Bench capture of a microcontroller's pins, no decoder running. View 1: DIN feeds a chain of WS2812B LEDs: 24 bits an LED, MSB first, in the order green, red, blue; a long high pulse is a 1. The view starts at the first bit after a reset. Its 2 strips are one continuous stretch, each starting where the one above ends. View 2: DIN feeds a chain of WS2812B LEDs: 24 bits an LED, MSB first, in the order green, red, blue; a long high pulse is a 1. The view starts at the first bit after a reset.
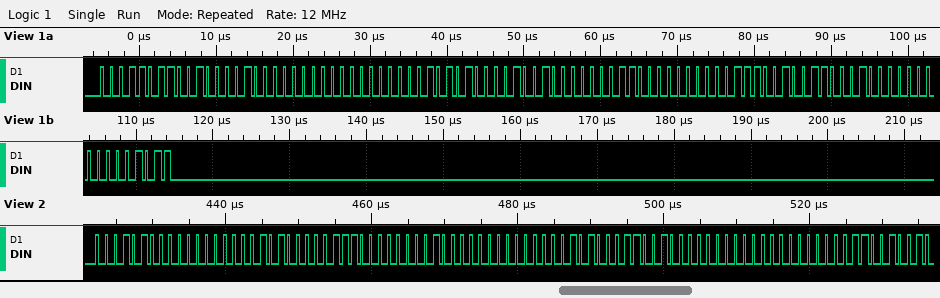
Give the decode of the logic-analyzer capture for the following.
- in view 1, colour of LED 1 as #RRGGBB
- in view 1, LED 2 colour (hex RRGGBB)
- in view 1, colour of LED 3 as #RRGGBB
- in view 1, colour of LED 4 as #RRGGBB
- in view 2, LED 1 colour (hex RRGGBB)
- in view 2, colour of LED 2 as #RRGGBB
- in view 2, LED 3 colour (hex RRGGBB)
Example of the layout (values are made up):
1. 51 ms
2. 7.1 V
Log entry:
1. #211B00
2. #2A0012
3. #000339
4. #00310B
5. #001428
6. #043800
7. #320A00
